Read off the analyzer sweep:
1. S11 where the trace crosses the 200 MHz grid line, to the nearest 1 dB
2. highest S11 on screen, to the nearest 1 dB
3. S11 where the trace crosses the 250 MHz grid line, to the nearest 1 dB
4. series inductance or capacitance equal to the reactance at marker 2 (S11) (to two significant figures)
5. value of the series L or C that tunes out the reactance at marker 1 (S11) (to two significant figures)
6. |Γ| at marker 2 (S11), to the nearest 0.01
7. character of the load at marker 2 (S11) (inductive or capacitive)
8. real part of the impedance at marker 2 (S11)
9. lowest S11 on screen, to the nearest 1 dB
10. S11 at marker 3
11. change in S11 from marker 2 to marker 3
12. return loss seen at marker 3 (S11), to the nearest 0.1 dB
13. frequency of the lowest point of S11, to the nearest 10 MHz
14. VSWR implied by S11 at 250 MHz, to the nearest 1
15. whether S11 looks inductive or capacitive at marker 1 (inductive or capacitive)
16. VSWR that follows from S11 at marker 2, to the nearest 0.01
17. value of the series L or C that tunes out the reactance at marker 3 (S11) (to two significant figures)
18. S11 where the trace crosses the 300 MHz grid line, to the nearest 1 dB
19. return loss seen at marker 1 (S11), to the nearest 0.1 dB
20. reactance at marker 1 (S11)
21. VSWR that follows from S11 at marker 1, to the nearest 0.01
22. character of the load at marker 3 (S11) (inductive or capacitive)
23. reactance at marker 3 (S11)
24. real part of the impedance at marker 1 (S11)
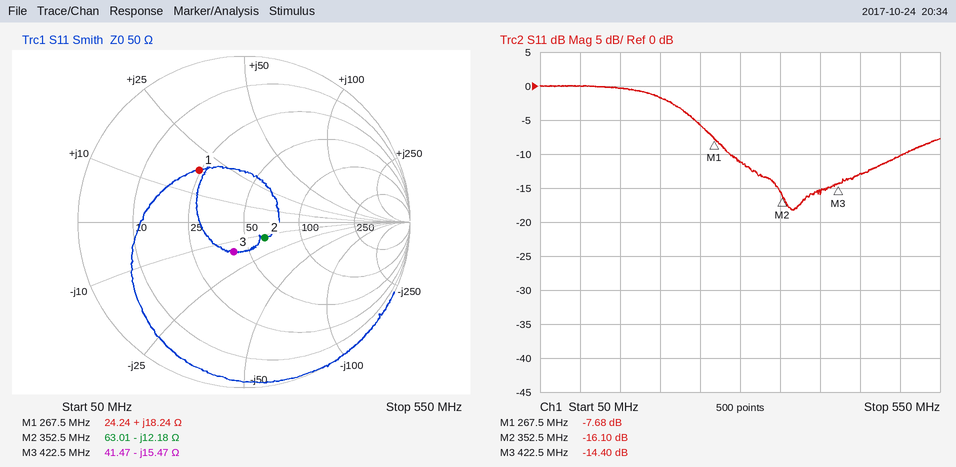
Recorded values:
-2 dB
0 dB
-6 dB
37 pF
33 pF
0.16
capacitive
63.01 Ω
-18 dB
-14.40 dB
1.70 dB
14.4 dB
370 MHz
3
inductive
1.37
5.8 nH
-11 dB
7.7 dB
+18.24 Ω
2.41
capacitive
-15.47 Ω
24.24 Ω
